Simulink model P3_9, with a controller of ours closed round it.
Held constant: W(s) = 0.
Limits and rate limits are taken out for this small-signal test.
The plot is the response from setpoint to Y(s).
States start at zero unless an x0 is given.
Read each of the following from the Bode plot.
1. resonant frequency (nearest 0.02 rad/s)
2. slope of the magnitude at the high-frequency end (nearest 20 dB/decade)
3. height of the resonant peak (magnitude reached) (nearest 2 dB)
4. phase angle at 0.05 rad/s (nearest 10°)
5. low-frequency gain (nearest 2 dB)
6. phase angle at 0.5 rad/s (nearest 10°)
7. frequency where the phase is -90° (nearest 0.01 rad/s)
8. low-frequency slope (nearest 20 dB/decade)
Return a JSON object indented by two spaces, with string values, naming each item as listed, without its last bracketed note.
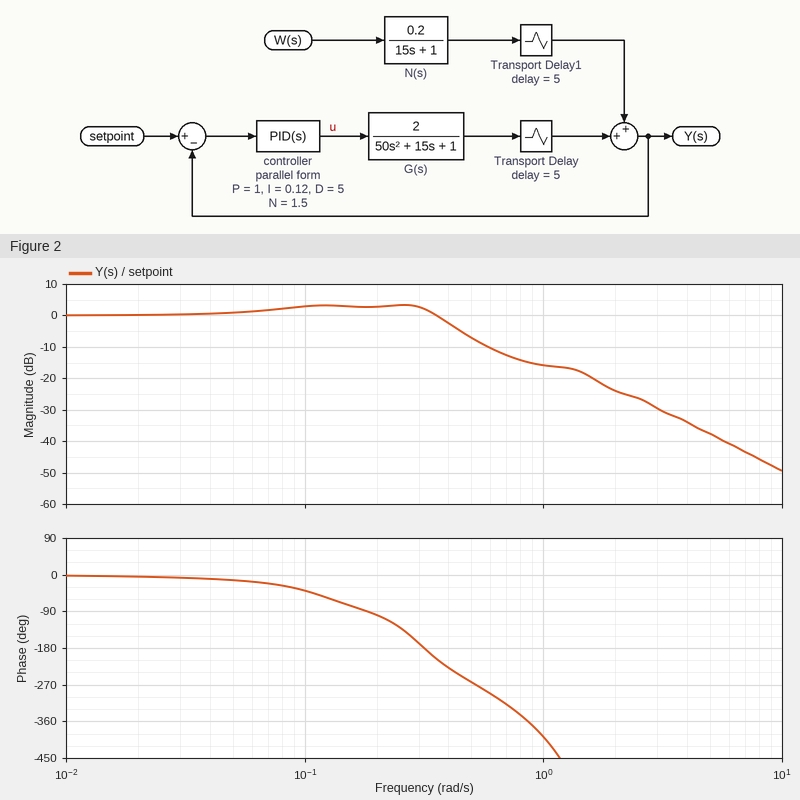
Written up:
{
  "resonant frequency": "0.26 rad/s",
  "slope of the magnitude at the high-frequency end": "-40 dB/decade",
  "height of the resonant peak (magnitude reached)": "4 dB",
  "phase angle at 0.05 rad/s": "-10°",
  "low-frequency gain": "0 dB",
  "phase angle at 0.5 rad/s": "-260°",
  "frequency where the phase is -90°": "0.18 rad/s",
  "low-frequency slope": "0 dB/decade"
}
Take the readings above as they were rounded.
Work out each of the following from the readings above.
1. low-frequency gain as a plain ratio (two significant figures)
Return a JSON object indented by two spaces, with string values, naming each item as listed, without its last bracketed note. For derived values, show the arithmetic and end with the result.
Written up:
{
  "low-frequency gain as a plain ratio": "10^(0 / 20) = 1.0"
}
